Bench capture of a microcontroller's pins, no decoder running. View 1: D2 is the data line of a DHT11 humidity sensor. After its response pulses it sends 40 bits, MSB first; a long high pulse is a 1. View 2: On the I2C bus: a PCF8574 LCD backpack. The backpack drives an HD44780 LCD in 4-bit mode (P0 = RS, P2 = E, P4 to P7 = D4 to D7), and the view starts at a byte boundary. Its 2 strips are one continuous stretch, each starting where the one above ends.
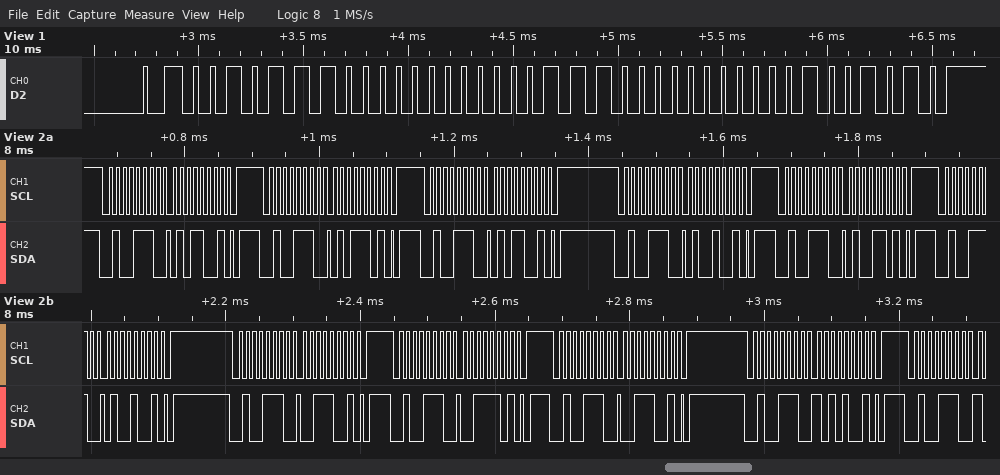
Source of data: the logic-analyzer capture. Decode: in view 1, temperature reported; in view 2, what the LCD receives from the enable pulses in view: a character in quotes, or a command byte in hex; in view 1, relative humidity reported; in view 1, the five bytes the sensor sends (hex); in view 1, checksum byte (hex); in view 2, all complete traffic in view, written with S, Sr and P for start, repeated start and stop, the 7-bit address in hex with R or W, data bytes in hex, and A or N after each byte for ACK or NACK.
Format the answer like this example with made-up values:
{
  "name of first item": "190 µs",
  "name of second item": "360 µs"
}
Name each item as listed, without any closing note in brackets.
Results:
{
  "in view 1, temperature reported": "28.0 °C",
  "in view 2, what the LCD receives from the enable pulses in view: a character in quotes, or a command byte in hex": "'T'",
  "in view 1, relative humidity reported": "46 %",
  "in view 1, the five bytes the sensor sends": "2E 00 1C 00 4A",
  "in view 1, checksum byte": "0x4A",
  "in view 2, all complete traffic in view, written with S, Sr and P for start, repeated start and stop, the 7-bit address in hex with R or W, data bytes in hex, and A or N after each byte for ACK or NACK": "S 27W A 59 A P S 27W A 5D A P S 27W A 59 A P S 27W A 49 A P S 27W A 4D A P S 27W A 49 A P S 27W A 39 A P S 27W A 3D A P S 27W A 39 A P S 27W A A9 A P S 27W A"
}
